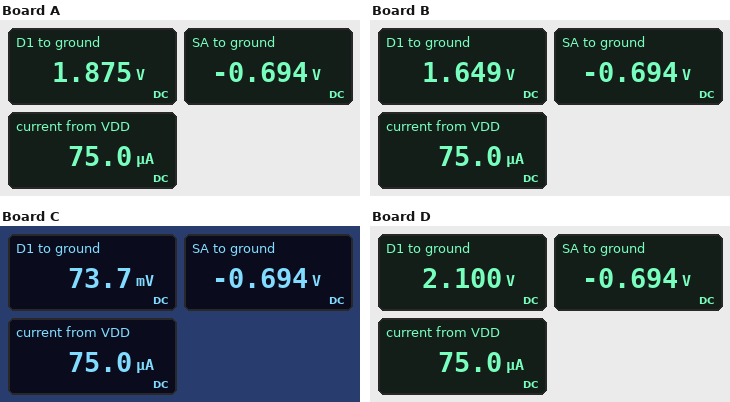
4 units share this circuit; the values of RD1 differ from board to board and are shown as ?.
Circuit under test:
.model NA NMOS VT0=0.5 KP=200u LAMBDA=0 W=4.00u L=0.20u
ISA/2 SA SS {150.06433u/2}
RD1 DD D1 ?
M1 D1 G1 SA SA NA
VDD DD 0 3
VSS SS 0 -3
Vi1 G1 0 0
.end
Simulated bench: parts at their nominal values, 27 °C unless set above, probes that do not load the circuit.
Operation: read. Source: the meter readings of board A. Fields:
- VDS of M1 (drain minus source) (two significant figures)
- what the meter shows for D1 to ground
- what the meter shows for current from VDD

2.6 V
1.875 V
75.0 µA
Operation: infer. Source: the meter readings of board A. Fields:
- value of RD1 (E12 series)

15 kΩ
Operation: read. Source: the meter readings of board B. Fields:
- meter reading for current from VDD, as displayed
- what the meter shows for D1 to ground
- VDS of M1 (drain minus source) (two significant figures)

75.0 µA
1.649 V
2.3 V
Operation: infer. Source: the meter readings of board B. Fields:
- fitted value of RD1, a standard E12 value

18 kΩ
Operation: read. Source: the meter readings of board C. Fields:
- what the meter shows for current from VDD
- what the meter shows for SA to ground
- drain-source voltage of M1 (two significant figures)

75.0 µA
-0.694 V
770 mV
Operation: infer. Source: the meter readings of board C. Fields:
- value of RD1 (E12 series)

39 kΩ
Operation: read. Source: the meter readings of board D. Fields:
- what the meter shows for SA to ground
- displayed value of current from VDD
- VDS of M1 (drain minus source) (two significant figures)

-0.694 V
75.0 µA
2.8 V
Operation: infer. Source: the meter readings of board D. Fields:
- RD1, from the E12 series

12 kΩ
